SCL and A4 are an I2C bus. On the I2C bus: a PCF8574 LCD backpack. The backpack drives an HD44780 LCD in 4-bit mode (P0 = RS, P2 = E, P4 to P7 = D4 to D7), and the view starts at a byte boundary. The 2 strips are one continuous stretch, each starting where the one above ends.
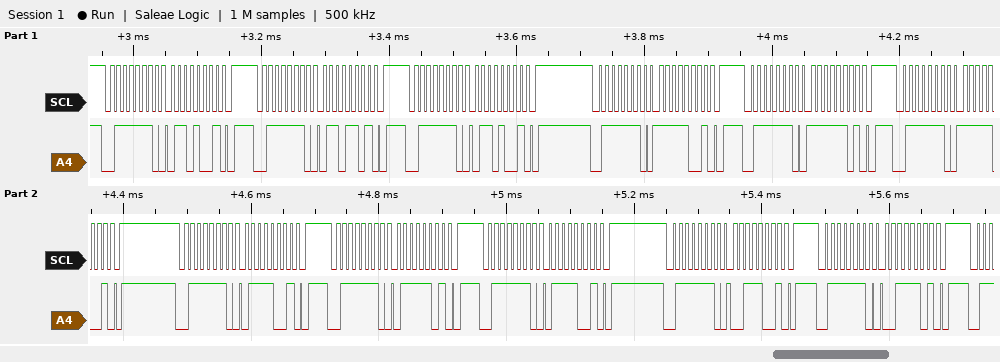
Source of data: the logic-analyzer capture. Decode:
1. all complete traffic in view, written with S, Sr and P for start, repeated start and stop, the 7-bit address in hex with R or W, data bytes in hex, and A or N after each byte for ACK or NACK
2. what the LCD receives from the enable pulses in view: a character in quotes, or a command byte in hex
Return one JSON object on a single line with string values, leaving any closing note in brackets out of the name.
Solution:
{"all complete traffic in view, written with S, Sr and P for start, repeated start and stop, the 7-bit address in hex with R or W, data bytes in hex, and A or N after each byte for ACK or NACK": "S 3FW A 69 A P S 3FW A 6D A P S 3FW A 69 A P S 3FW A F9 A P S 3FW A FD A P S 3FW A F9 A P S 3FW A 79 A P S 3FW A 7D A P S 3FW A 79 A P S 3FW A 39 A P S 3FW A 3D A P", "what the LCD receives from the enable pulses in view: a character in quotes, or a command byte in hex": "'o'"}
